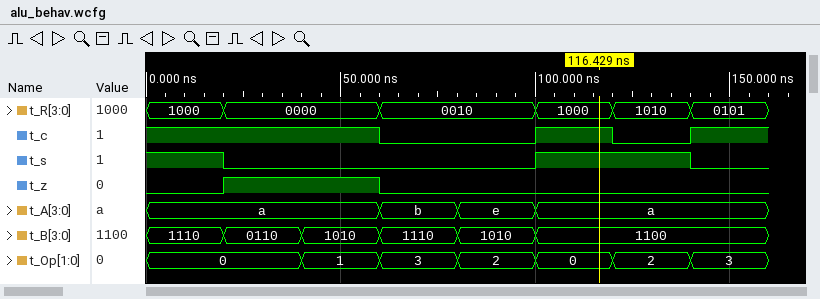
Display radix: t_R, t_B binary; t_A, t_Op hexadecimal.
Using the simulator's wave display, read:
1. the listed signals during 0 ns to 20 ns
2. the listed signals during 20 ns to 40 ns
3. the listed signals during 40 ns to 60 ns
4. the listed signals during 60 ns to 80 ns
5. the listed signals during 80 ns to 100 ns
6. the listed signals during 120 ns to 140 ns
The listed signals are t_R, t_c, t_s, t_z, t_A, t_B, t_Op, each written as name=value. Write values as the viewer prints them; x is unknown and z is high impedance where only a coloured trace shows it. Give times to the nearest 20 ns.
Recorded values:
t_R=1000, t_c=1, t_s=1, t_z=0, t_A=a, t_B=1110, t_Op=0
t_R=0000, t_c=1, t_s=0, t_z=1, t_A=a, t_B=0110, t_Op=0
t_R=0000, t_c=1, t_s=0, t_z=1, t_A=a, t_B=1010, t_Op=1
t_R=0010, t_c=0, t_s=0, t_z=0, t_A=b, t_B=1110, t_Op=3
t_R=0010, t_c=0, t_s=0, t_z=0, t_A=e, t_B=1010, t_Op=2
t_R=1010, t_c=0, t_s=1, t_z=0, t_A=a, t_B=1100, t_Op=2
